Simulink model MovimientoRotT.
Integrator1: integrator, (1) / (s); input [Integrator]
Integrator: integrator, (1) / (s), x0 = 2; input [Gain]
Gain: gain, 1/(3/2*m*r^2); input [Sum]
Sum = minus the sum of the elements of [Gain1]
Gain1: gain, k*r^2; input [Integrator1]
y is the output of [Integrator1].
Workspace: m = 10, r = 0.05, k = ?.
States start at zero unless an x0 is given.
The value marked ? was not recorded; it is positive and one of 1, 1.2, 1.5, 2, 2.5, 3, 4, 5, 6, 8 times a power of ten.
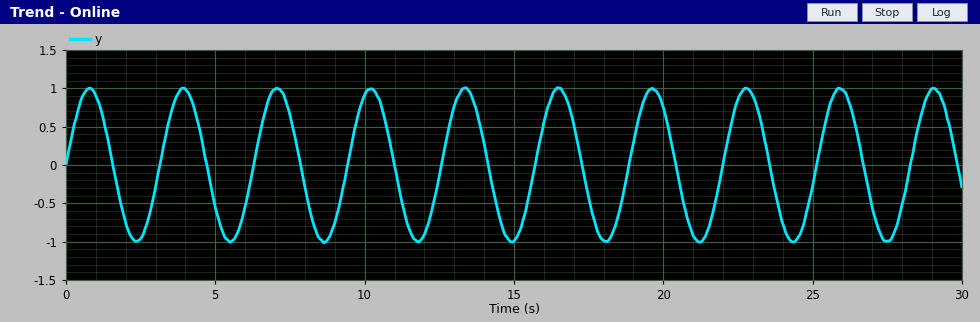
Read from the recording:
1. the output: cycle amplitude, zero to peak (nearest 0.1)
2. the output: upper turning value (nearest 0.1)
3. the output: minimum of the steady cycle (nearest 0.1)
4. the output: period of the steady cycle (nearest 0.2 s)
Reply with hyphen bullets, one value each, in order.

- 1.0
- 1.0
- -1.0
- 3.2 s
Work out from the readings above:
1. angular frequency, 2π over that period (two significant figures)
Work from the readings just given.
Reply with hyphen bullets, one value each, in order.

- 2.0 rad/s
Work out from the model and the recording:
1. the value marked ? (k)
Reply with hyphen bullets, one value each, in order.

- 60
